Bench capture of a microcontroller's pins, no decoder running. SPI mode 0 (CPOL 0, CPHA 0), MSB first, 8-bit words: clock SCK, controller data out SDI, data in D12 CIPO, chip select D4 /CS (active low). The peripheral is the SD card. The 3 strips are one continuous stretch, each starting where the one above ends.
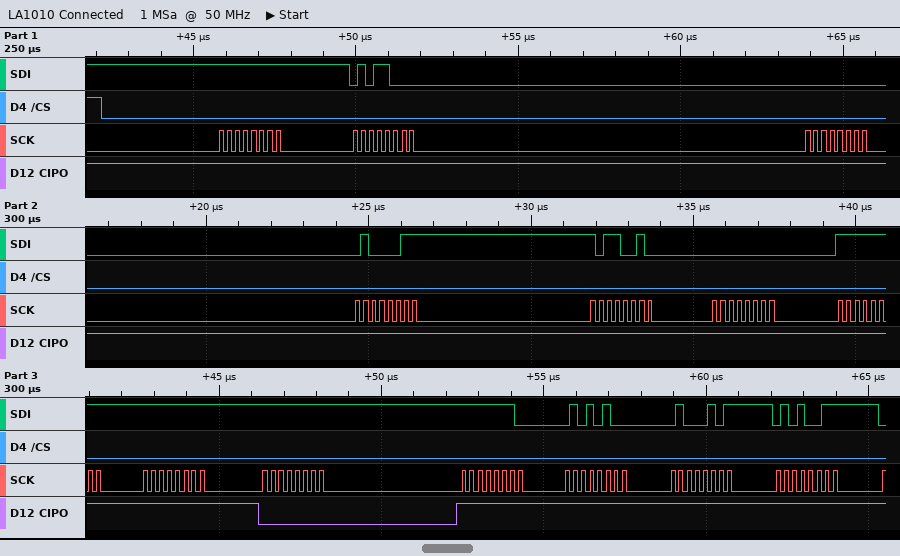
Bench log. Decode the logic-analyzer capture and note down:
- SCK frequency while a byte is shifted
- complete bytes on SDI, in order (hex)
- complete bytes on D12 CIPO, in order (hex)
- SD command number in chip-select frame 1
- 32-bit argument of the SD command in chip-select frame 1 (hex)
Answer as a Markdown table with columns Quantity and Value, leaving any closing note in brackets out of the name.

| Quantity | Value |
|---|---|
| SCK frequency while a byte is shifted | 4 MHz |
| complete bytes on SDI, in order | 0xFF 0x58 0x00 0x43 0xB2 0x00 0xFF 0xFF 0xFF 0xFE 0x54 0x45 0x53 |
| complete bytes on D12 CIPO, in order | 0xFF 0xFF 0xFF 0xFF 0xFF 0xFF 0xFF 0xFF 0x00 0xFF 0xFF 0xFF 0xFF |
| SD command number in chip-select frame 1 | CMD24 |
| 32-bit argument of the SD command in chip-select frame 1 | 0x0043B200 |
